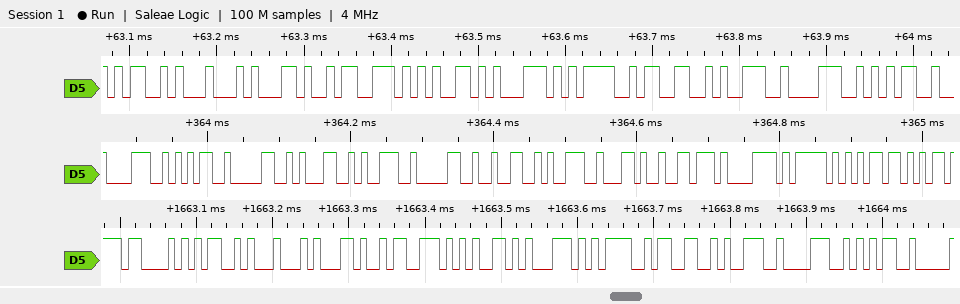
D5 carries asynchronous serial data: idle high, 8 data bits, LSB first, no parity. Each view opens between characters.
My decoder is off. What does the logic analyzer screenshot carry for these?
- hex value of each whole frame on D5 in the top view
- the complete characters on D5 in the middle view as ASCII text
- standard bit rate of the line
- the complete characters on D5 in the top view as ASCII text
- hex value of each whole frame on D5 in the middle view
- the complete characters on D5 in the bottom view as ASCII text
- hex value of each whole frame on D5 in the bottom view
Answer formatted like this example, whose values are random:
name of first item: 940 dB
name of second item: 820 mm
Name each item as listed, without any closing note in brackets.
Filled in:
hex value of each whole frame on D5 in the top view: 4D, 44, 2C, 73, 65, 71, 3D, 33, 39, 38, 35
the complete characters on D5 in the middle view as ASCII text: "85019029,vx_m"
standard bit rate of the line: 115200 baud
the complete characters on D5 in the top view as ASCII text: "MD,seq=3985"
hex value of each whole frame on D5 in the middle view: 38, 35, 30, 31, 39, 30, 32, 39, 2C, 76, 78, 5F, 6D
the complete characters on D5 in the bottom view as ASCII text: "CMD,seq=3985"
hex value of each whole frame on D5 in the bottom view: 43, 4D, 44, 2C, 73, 65, 71, 3D, 33, 39, 38, 35
